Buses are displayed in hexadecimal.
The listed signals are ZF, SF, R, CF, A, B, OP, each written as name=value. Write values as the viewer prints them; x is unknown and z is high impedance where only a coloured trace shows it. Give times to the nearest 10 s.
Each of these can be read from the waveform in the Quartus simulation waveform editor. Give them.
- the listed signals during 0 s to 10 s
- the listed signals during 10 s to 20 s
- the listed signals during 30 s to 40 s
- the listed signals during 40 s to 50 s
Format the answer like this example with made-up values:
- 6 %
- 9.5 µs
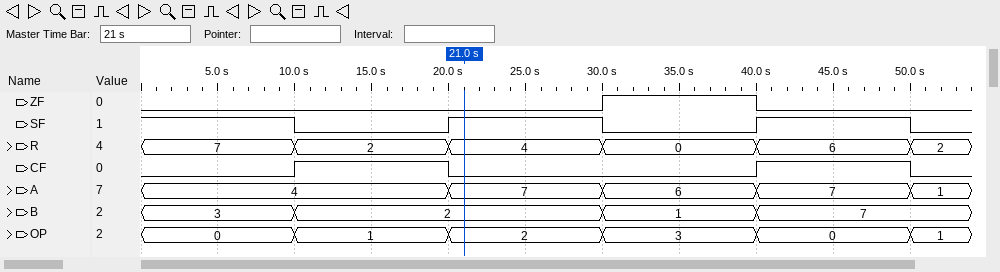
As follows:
- ZF=0, SF=1, R=7, CF=0, A=4, B=3, OP=0
- ZF=0, SF=0, R=2, CF=1, A=4, B=2, OP=1
- ZF=1, SF=0, R=0, CF=0, A=6, B=1, OP=3
- ZF=0, SF=1, R=6, CF=1, A=7, B=7, OP=0
